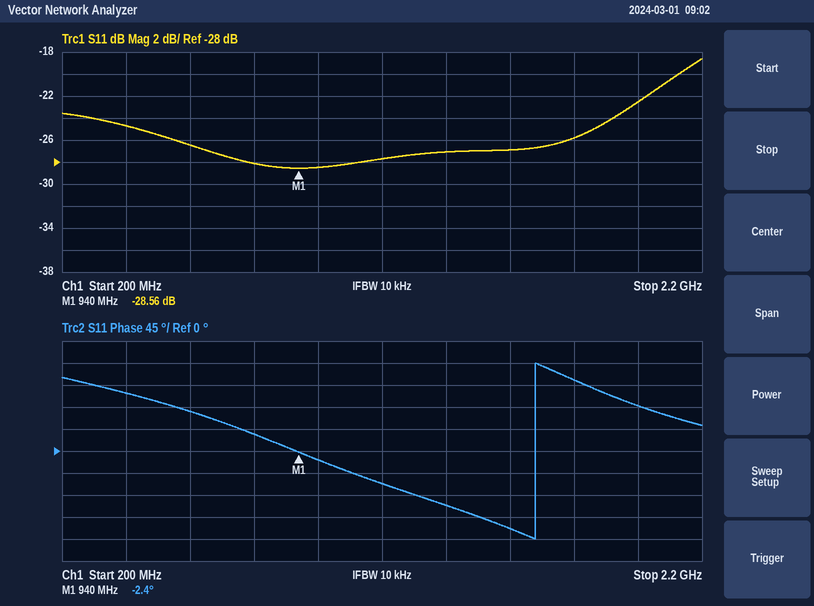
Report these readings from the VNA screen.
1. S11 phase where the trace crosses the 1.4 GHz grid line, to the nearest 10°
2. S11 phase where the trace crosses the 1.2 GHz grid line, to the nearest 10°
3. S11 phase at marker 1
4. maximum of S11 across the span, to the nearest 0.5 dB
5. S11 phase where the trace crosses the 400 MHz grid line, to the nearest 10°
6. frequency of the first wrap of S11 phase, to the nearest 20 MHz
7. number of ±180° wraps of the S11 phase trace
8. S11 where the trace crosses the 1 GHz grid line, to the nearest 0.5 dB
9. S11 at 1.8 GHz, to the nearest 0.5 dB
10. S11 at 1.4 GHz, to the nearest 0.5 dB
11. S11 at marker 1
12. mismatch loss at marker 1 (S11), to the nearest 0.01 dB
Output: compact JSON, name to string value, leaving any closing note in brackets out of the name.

{"S11 phase where the trace crosses the 1.4 GHz grid line, to the nearest 10°": "-110°", "S11 phase where the trace crosses the 1.2 GHz grid line, to the nearest 10°": "-70°", "S11 phase at marker 1": "-2.4°", "maximum of S11 across the span, to the nearest 0.5 dB": "-18.5 dB", "S11 phase where the trace crosses the 400 MHz grid line, to the nearest 10°": "120°", "frequency of the first wrap of S11 phase, to the nearest 20 MHz": "1.68 GHz", "number of ±180° wraps of the S11 phase trace": "1", "S11 where the trace crosses the 1 GHz grid line, to the nearest 0.5 dB": "-28.5 dB", "S11 at 1.8 GHz, to the nearest 0.5 dB": "-26.0 dB", "S11 at 1.4 GHz, to the nearest 0.5 dB": "-27.0 dB", "S11 at marker 1": "-28.56 dB", "mismatch loss at marker 1 (S11), to the nearest 0.01 dB": "0.01 dB"}
